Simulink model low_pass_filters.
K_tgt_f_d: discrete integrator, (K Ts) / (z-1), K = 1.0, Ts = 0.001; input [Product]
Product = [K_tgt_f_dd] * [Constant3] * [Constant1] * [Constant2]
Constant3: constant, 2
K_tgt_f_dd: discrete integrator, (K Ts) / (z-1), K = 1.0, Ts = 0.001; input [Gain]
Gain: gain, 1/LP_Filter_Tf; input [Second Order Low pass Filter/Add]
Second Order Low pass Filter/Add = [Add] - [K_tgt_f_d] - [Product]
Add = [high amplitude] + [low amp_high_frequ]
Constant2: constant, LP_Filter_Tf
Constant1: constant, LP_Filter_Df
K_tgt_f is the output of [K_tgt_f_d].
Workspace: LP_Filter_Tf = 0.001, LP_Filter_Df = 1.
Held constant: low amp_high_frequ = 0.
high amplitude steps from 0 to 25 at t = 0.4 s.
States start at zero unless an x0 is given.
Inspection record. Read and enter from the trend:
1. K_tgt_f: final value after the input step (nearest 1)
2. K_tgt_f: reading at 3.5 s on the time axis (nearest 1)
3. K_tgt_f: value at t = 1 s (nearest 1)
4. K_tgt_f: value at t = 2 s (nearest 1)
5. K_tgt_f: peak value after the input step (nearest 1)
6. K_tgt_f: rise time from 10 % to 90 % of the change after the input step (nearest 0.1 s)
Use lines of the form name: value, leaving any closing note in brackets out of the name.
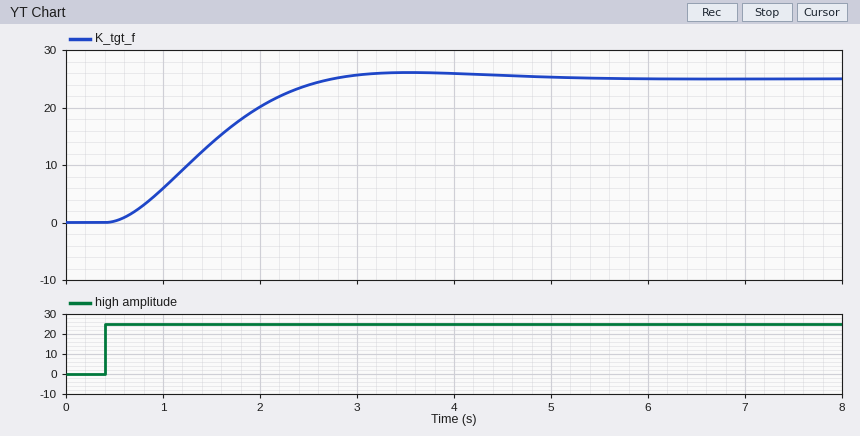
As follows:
K_tgt_f: final value after the input step: 25
K_tgt_f: reading at 3.5 s on the time axis: 26
K_tgt_f: value at t = 1 s: 6
K_tgt_f: value at t = 2 s: 20
K_tgt_f: peak value after the input step: 26
K_tgt_f: rise time from 10 % to 90 % of the change after the input step: 1.5 s
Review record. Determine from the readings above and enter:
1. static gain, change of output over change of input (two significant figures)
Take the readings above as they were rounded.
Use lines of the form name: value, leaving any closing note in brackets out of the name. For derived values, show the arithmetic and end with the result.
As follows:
static gain, change of output over change of input: (25 - 0) / (25 - 0) = 1.0
